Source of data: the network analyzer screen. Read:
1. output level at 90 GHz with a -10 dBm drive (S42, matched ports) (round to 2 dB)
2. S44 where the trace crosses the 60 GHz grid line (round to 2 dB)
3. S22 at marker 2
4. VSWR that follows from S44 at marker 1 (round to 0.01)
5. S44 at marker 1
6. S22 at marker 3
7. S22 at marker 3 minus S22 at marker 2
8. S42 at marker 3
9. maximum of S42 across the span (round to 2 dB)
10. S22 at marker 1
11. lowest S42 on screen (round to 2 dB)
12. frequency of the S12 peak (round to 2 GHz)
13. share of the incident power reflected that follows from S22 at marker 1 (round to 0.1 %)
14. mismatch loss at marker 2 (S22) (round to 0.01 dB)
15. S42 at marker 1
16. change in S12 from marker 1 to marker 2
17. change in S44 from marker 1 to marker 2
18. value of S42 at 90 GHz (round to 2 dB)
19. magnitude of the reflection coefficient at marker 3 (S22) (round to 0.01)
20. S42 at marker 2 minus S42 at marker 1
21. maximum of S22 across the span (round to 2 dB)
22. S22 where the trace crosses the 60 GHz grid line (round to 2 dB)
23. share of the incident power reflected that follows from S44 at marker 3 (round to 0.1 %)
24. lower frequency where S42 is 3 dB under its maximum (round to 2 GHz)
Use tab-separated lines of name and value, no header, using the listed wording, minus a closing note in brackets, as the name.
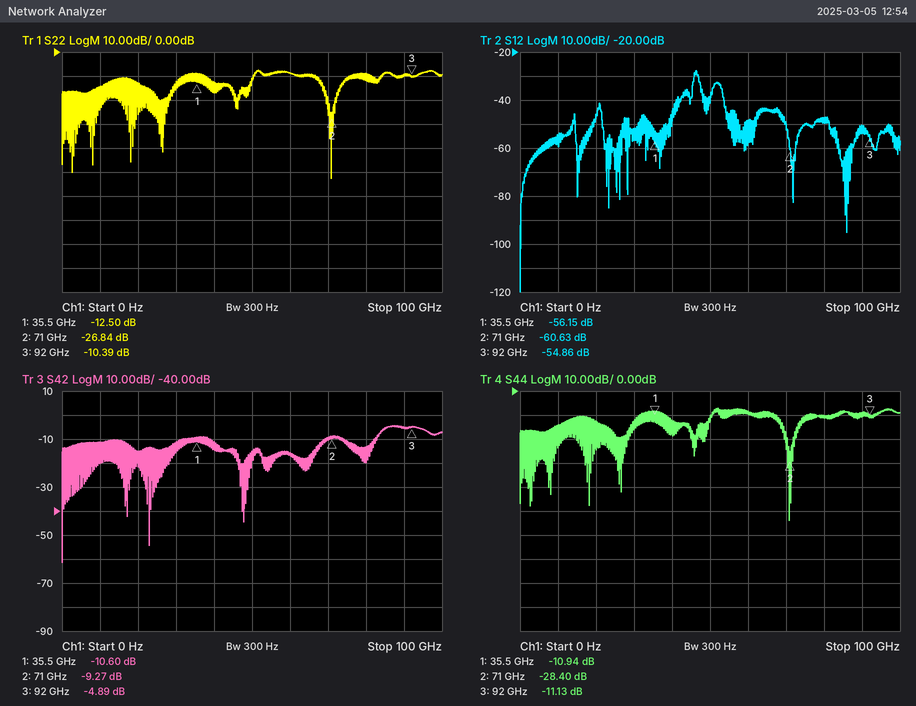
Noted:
output level at 90 GHz with a -10 dBm drive (S42, matched ports)	-16 dBm
S44 where the trace crosses the 60 GHz grid line	-8 dB
S22 at marker 2	-26.84 dB
VSWR that follows from S44 at marker 1	1.79
S44 at marker 1	-10.94 dB
S22 at marker 3	-10.39 dB
S22 at marker 3 minus S22 at marker 2	16.45 dB
S42 at marker 3	-4.89 dB
maximum of S42 across the span	-4 dB
S22 at marker 1	-12.50 dB
lowest S42 on screen	-62 dB
frequency of the S12 peak	46 GHz
share of the incident power reflected that follows from S22 at marker 1	5.6 %
mismatch loss at marker 2 (S22)	0.01 dB
S42 at marker 1	-10.60 dB
change in S12 from marker 1 to marker 2	-4.48 dB
change in S44 from marker 1 to marker 2	-17.46 dB
value of S42 at 90 GHz	-6 dB
magnitude of the reflection coefficient at marker 3 (S22)	0.30
S42 at marker 2 minus S42 at marker 1	1.33 dB
maximum of S22 across the span	-8 dB
S22 where the trace crosses the 60 GHz grid line	-8 dB
share of the incident power reflected that follows from S44 at marker 3	7.7 %
lower frequency where S42 is 3 dB under its maximum	84 GHz
